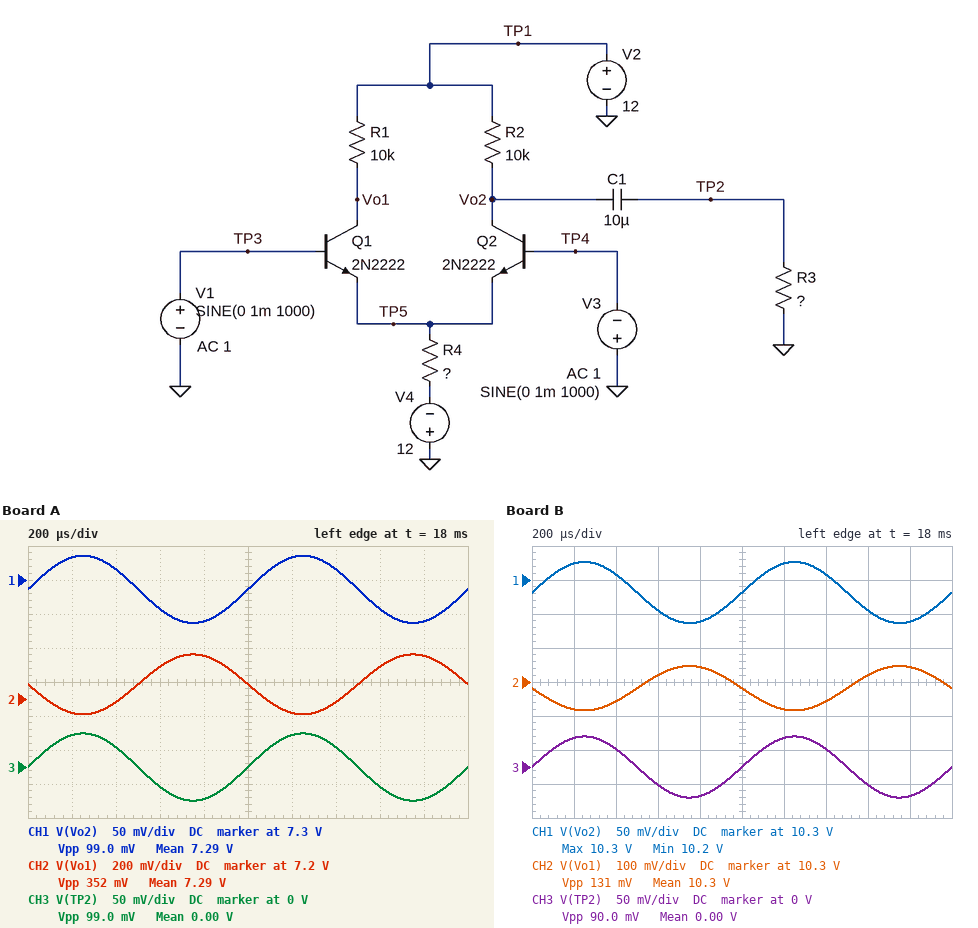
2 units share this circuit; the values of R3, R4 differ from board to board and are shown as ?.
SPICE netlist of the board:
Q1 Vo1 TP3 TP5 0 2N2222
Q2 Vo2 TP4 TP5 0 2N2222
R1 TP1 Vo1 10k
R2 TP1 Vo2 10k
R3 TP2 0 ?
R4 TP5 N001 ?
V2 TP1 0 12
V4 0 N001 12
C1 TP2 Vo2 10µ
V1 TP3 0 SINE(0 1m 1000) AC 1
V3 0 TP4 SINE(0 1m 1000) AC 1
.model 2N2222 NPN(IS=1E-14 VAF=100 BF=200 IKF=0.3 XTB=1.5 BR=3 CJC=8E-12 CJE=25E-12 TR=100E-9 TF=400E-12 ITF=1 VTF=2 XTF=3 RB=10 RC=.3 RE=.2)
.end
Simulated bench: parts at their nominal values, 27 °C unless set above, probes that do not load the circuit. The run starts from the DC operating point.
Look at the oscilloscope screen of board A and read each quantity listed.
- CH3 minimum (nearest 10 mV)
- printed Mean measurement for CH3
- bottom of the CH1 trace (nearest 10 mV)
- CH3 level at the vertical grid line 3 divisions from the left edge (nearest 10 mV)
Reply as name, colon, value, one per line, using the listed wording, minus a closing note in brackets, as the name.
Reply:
CH3 minimum: -50 mV
printed Mean measurement for CH3: 0.00 V
bottom of the CH1 trace: 7.24 V
CH3 level at the vertical grid line 3 divisions from the left edge: -30 mV
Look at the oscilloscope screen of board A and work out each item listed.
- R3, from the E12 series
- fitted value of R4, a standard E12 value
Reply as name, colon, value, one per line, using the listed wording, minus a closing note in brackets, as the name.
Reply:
R3, from the E12 series: 3.9 kΩ
fitted value of R4, a standard E12 value: 12 kΩ
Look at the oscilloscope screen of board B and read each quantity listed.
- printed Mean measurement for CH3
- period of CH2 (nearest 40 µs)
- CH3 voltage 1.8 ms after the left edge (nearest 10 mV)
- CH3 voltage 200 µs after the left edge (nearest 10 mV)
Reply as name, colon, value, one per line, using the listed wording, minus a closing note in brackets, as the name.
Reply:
printed Mean measurement for CH3: 0.00 V
period of CH2: 1.00 ms
CH3 voltage 1.8 ms after the left edge: -40 mV
CH3 voltage 200 µs after the left edge: 40 mV
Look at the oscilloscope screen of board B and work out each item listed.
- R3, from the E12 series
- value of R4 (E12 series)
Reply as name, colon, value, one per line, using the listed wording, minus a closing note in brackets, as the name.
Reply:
R3, from the E12 series: 22 kΩ
value of R4: 33 kΩ
